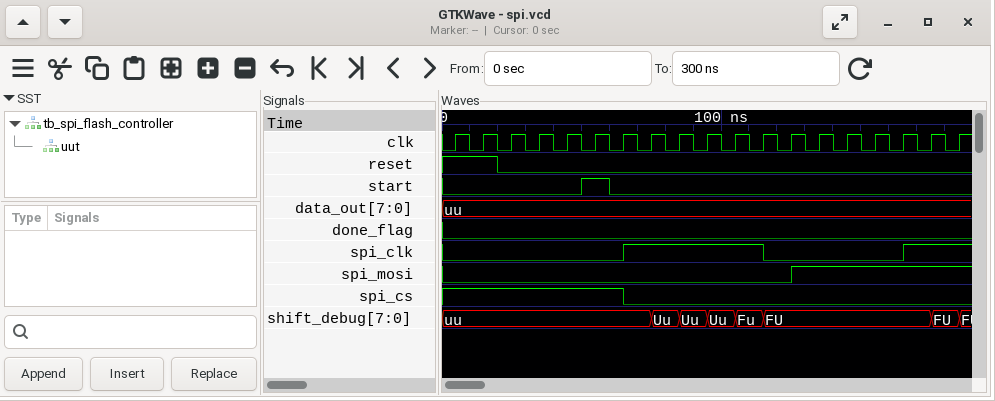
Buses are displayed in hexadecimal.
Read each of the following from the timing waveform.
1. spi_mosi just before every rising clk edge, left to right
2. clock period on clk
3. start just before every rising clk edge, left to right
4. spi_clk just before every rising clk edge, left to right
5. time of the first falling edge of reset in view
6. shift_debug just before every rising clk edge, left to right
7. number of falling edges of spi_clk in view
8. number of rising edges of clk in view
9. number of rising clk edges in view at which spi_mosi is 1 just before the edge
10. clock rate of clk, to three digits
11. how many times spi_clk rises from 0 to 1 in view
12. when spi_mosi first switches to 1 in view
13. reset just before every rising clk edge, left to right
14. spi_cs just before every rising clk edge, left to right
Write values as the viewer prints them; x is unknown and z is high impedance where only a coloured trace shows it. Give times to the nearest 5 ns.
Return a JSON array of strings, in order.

["0 0 0 0 0 0 0 0 0 0 0 0 0 1 1 1 1 1 1", "10 ns", "0 0 0 0 0 1 0 0 0 0 0 0 0 0 0 0 0 0 0", "0 0 0 0 0 0 0 1 1 1 1 1 0 0 0 0 0 1 1", "20 ns", "uu, uu, uu, uu, uu, uu, uu, uu, Uu, Uu, Uu, Fu, FU, FU, FU, FU, FU, FU, FU", "1", "19", "6", "100 MHz", "2", "125 ns", "1 1 0 0 0 0 0 0 0 0 0 0 0 0 0 0 0 0 0", "1 1 1 1 1 1 1 0 0 0 0 0 0 0 0 0 0 0 0"]
